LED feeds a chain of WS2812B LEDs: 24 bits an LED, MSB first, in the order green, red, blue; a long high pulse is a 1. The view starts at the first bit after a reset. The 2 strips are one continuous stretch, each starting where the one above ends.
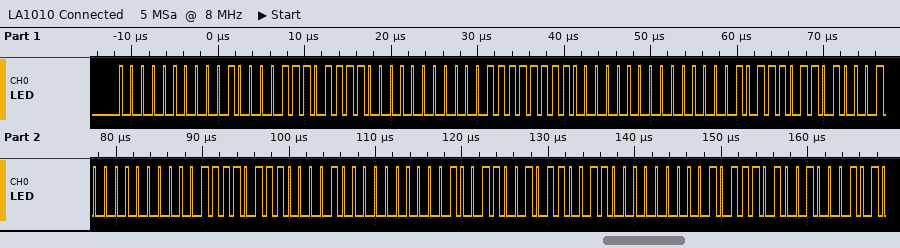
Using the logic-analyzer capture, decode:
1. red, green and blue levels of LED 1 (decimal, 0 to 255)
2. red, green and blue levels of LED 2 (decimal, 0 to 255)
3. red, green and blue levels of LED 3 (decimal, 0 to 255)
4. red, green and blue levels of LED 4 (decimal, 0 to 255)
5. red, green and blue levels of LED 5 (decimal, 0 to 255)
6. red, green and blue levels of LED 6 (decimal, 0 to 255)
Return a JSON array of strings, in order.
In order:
["33, 0, 222", "63, 0, 192", "93, 0, 162", "123, 0, 132", "153, 0, 102", "186, 0, 69"]
